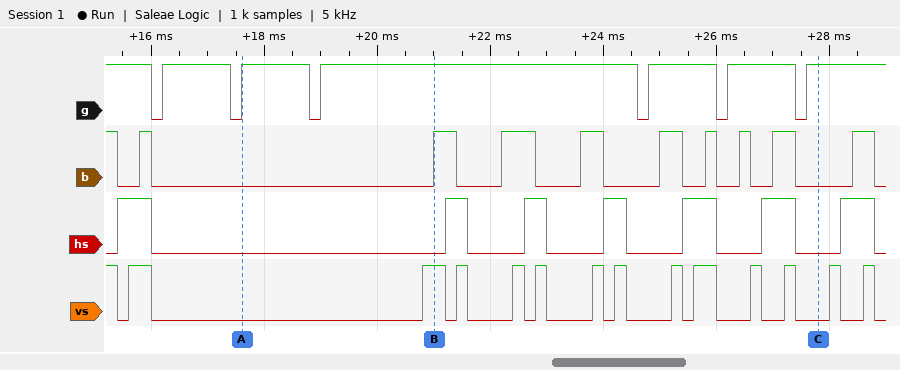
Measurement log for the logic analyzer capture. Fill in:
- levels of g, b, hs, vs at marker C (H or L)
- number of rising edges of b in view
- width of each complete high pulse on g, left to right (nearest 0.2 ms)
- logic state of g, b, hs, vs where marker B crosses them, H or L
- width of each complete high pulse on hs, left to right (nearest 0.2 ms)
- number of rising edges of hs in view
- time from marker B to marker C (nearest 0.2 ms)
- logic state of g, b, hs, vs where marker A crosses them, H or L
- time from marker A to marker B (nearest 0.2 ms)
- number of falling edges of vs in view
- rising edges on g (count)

g=H, b=L, hs=L, vs=L
9
1.2 ms, 1.2 ms, 5.6 ms, 1.2 ms, 1.2 ms
g=H, b=H, hs=L, vs=H
0.6 ms, 0.4 ms, 0.4 ms, 0.4 ms, 0.6 ms, 0.6 ms, 0.6 ms
7
6.8 ms
g=H, b=L, hs=L, vs=L
3.4 ms
14
6
